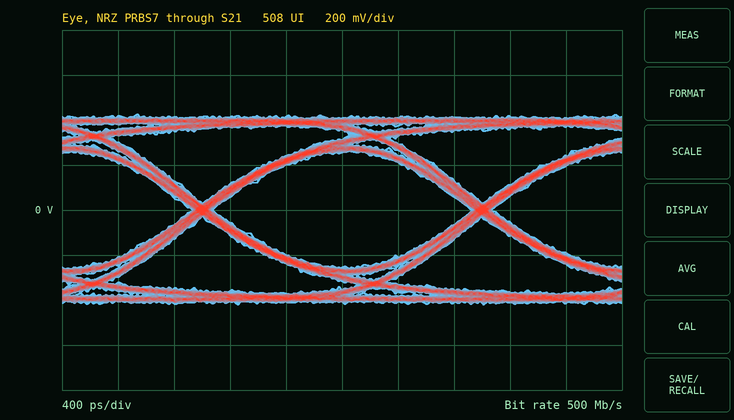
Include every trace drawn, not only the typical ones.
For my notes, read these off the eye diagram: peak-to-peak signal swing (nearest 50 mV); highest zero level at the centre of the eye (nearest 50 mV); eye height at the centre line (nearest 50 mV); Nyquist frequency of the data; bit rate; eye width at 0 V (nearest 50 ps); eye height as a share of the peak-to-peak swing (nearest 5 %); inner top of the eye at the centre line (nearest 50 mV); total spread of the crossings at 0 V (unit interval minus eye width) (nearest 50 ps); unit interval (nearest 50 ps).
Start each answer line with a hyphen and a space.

- 850 mV
- -250 mV
- 500 mV
- 250 MHz
- 500 Mb/s
- 1.85 ns
- 60 %
- 250 mV
- 150 ps
- 2.00 ns
